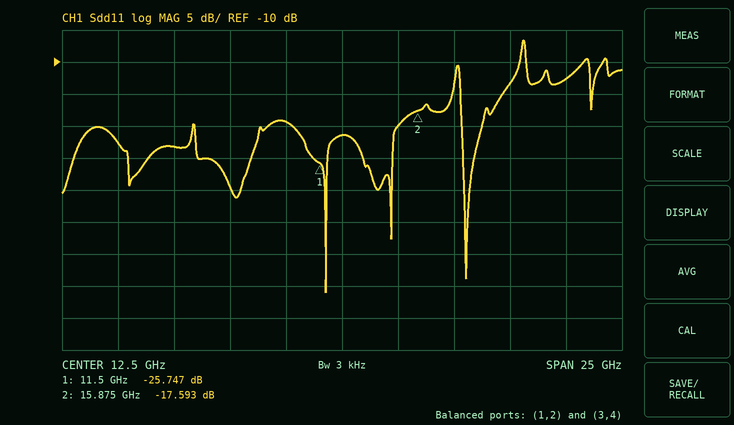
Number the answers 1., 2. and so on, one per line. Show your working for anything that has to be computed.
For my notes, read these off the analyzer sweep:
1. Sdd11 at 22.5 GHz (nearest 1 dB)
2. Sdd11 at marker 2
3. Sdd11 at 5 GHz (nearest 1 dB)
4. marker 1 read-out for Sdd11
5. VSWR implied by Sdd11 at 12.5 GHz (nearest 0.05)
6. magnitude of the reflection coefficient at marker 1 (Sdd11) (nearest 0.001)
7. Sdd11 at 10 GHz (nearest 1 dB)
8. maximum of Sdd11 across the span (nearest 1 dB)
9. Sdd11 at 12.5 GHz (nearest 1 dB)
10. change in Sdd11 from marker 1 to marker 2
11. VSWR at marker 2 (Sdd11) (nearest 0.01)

1. -13 dB
2. -17.593 dB
3. -23 dB
4. -25.747 dB
5. |Γ| = 10^(-21/20) = 0.0891; VSWR = (1 + 0.0891)/(1 − 0.0891) ≈ 1.20
6. 10^(-25.747/20) ≈ 0.052
7. -19 dB
8. -7 dB
9. -21 dB
10. -17.593 − (-25.747) = 8.154 dB
11. (1 + 0.1319)/(1 − 0.1319) ≈ 1.30
